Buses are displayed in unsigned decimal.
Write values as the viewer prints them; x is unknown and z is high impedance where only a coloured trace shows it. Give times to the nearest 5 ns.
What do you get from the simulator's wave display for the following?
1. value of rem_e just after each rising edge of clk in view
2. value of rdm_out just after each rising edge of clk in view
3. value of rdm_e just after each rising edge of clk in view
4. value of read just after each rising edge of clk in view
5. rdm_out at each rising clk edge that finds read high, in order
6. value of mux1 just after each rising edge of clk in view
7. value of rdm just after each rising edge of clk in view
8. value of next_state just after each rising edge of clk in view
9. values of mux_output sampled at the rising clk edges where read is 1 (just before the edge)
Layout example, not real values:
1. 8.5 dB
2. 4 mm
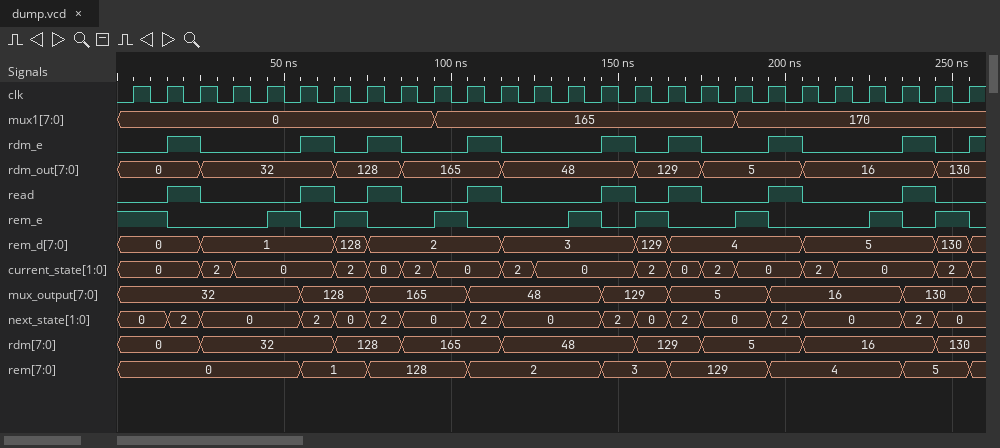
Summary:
1. 1 0 0 0 1 0 1 0 0 1 0 0 0 1 0 1 0 0 1 0 0 0 1 0 1 0
2. 0, 0, 32, 32, 32, 32, 128, 128, 165, 165, 165, 48, 48, 48, 48, 129, 129, 5, 5, 5, 16, 16, 16, 16, 130, 130
3. 0 1 0 0 0 1 0 1 0 0 1 0 0 0 1 0 1 0 0 1 0 0 0 1 0 1
4. 0 1 0 0 0 1 0 1 0 0 1 0 0 0 1 0 1 0 0 1 0 0 0 1 0 0
5. 0, 32, 128, 165, 48, 129, 5, 16
6. 0, 0, 0, 0, 0, 0, 0, 0, 0, 165, 165, 165, 165, 165, 165, 165, 165, 165, 170, 170, 170, 170, 170, 170, 170, 170
7. 0, 0, 32, 32, 32, 32, 128, 128, 165, 165, 165, 48, 48, 48, 48, 129, 129, 5, 5, 5, 16, 16, 16, 16, 130, 130
8. 0, 2, 0, 0, 0, 2, 0, 2, 0, 0, 2, 0, 0, 0, 2, 0, 2, 0, 0, 2, 0, 0, 0, 2, 0, 0
9. 32, 128, 165, 48, 129, 5, 16, 130
